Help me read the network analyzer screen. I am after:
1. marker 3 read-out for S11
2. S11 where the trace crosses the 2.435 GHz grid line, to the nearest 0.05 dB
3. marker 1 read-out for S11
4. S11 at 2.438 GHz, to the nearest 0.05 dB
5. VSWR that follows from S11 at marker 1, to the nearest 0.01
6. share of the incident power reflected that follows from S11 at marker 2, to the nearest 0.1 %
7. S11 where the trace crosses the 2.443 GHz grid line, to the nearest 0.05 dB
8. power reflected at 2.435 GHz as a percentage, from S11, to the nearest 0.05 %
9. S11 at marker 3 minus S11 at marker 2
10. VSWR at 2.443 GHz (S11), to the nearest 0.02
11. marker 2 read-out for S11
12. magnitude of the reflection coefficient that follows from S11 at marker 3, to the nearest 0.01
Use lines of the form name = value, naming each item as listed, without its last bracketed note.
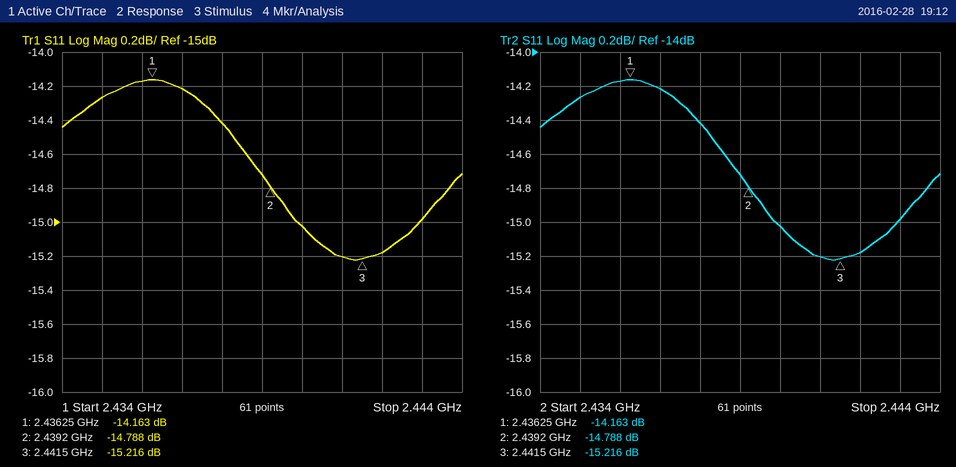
marker 3 read-out for S11 = -15.216 dB
S11 where the trace crosses the 2.435 GHz grid line, to the nearest 0.05 dB = -14.25 dB
marker 1 read-out for S11 = -14.163 dB
S11 at 2.438 GHz, to the nearest 0.05 dB = -14.40 dB
VSWR that follows from S11 at marker 1, to the nearest 0.01 = 1.49
share of the incident power reflected that follows from S11 at marker 2, to the nearest 0.1 % = 3.3 %
S11 where the trace crosses the 2.443 GHz grid line, to the nearest 0.05 dB = -15.00 dB
power reflected at 2.435 GHz as a percentage, from S11, to the nearest 0.05 % = 3.75 %
S11 at marker 3 minus S11 at marker 2 = -0.428 dB
VSWR at 2.443 GHz (S11), to the nearest 0.02 = 1.44
marker 2 read-out for S11 = -14.788 dB
magnitude of the reflection coefficient that follows from S11 at marker 3, to the nearest 0.01 = 0.17
